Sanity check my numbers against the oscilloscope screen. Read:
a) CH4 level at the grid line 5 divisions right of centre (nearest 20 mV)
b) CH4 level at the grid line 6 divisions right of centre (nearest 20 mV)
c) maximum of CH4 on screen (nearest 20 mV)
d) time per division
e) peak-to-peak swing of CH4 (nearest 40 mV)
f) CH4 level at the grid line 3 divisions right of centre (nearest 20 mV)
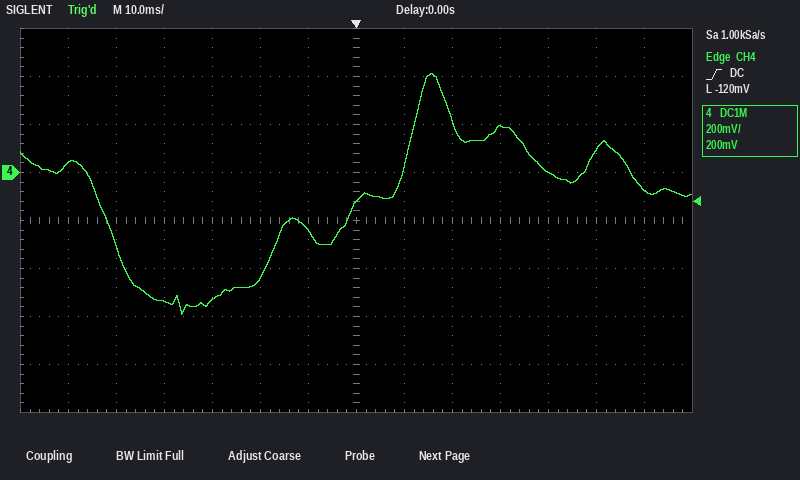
100 mV
-80 mV
420 mV
10 ms
1.00 V
200 mV
